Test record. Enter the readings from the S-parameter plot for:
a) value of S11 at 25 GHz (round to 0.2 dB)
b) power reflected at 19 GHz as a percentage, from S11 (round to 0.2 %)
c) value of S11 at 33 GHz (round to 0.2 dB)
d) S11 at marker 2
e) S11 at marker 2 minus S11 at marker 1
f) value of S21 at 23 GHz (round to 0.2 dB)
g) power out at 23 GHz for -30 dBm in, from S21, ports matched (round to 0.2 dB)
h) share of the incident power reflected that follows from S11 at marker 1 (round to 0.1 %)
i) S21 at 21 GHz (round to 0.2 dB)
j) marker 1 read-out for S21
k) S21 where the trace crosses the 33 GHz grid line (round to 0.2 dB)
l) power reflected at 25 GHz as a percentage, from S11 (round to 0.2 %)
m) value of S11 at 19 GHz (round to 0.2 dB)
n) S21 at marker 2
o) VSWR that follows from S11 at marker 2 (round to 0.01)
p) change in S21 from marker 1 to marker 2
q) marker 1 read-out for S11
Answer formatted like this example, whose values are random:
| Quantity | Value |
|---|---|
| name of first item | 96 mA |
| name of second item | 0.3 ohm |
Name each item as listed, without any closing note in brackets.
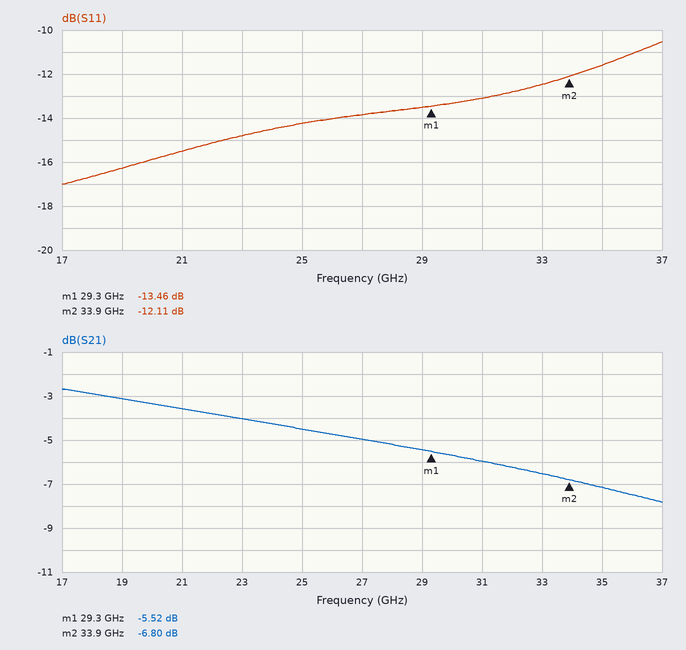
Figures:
| Quantity | Value |
|---|---|
| value of S11 at 25 GHz | -14.2 dB |
| power reflected at 19 GHz as a percentage, from S11 | 2.4 % |
| value of S11 at 33 GHz | -12.4 dB |
| S11 at marker 2 | -12.11 dB |
| S11 at marker 2 minus S11 at marker 1 | 1.35 dB |
| value of S21 at 23 GHz | -4.0 dB |
| power out at 23 GHz for -30 dBm in, from S21, ports matched | -34.0 dBm |
| share of the incident power reflected that follows from S11 at marker 1 | 4.5 % |
| S21 at 21 GHz | -3.6 dB |
| marker 1 read-out for S21 | -5.52 dB |
| S21 where the trace crosses the 33 GHz grid line | -6.6 dB |
| power reflected at 25 GHz as a percentage, from S11 | 3.8 % |
| value of S11 at 19 GHz | -16.2 dB |
| S21 at marker 2 | -6.80 dB |
| VSWR that follows from S11 at marker 2 | 1.66 |
| change in S21 from marker 1 to marker 2 | -1.28 dB |
| marker 1 read-out for S11 | -13.46 dB |
